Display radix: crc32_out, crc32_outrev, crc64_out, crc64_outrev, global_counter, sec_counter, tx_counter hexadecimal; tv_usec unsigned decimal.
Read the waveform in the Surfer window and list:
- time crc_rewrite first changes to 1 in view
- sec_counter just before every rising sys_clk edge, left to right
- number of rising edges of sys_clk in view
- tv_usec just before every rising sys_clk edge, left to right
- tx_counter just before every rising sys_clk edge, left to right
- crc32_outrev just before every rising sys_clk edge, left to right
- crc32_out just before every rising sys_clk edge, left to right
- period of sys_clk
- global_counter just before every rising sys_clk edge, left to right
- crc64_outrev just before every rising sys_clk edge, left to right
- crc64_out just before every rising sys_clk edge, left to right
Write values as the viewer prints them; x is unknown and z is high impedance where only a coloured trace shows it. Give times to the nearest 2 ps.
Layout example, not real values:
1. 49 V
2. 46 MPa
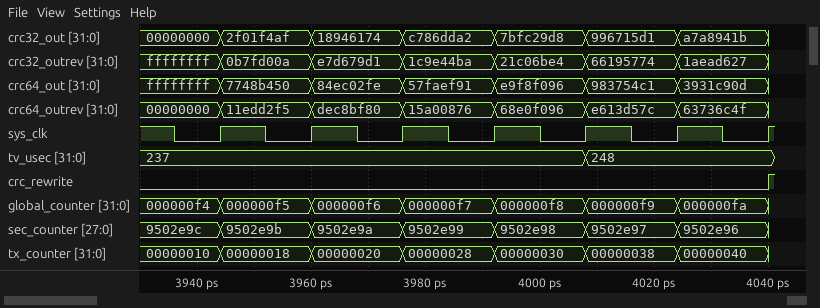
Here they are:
1. 4040 ps
2. 9502e9c, 9502e9b, 9502e9a, 9502e99, 9502e98, 9502e97, 9502e96
3. 7
4. 237, 237, 237, 237, 237, 248, 248
5. 00000010, 00000018, 00000020, 00000028, 00000030, 00000038, 00000040
6. ffffffff, 0b7fd00a, e7d679d1, 1c9e44ba, 21c06be4, 66195774, 1aead627
7. 00000000, 2f01f4af, 18946174, c786dda2, 7bfc29d8, 996715d1, a7a8941b
8. 16 ps
9. 000000f4, 000000f5, 000000f6, 000000f7, 000000f8, 000000f9, 000000fa
10. 00000000, 11edd2f5, dec8bf80, 15a00876, 68e0f096, e613d57c, 63736c4f
11. ffffffff, 7748b450, 84ec02fe, 57faef91, e9f8f096, 983754c1, 3931c90d
